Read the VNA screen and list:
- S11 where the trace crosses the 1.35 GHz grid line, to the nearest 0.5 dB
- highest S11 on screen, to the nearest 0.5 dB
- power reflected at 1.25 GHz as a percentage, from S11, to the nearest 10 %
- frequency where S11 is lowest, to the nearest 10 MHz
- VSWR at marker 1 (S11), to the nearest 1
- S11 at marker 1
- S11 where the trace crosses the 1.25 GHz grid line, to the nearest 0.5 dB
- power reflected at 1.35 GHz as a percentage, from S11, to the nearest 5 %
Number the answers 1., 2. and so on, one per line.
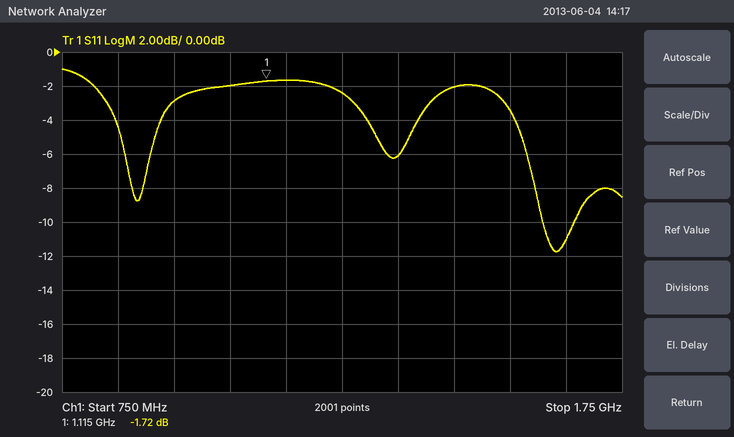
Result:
1. -6.0 dB
2. -1.0 dB
3. 60 %
4. 1.63 GHz
5. 10
6. -1.72 dB
7. -2.5 dB
8. 25 %
